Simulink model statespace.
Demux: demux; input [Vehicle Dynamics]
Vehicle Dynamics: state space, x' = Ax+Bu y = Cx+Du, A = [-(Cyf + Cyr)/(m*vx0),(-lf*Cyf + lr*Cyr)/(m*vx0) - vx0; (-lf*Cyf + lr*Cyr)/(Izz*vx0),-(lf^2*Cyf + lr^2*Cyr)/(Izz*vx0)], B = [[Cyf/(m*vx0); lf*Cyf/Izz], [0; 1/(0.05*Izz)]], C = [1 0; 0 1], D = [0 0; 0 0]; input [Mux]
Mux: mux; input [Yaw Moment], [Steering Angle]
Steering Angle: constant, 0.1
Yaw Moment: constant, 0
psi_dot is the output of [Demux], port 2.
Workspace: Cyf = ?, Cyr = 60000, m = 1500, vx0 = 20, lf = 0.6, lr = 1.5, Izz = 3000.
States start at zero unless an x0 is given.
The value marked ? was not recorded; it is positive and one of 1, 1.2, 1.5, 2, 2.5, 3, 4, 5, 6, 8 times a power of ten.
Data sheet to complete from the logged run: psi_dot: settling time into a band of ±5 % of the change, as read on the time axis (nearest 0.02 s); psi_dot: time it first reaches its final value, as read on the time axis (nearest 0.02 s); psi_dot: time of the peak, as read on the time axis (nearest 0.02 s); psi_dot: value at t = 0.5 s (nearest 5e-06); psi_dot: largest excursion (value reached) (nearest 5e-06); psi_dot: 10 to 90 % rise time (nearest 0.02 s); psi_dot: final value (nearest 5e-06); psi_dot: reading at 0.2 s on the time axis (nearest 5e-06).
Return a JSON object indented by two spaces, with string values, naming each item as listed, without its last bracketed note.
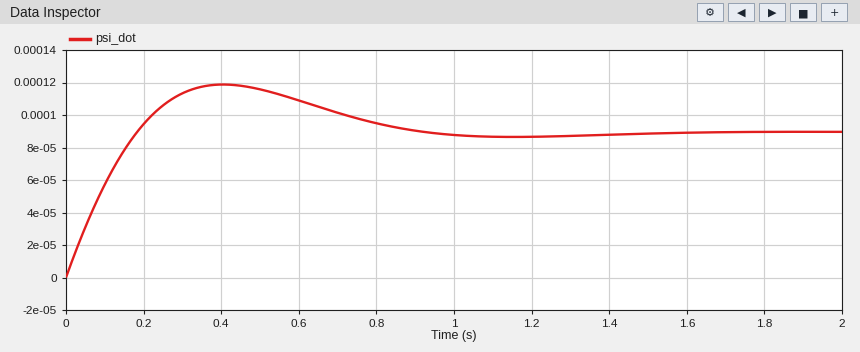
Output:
{
  "psi_dot: settling time into a band of ±5 % of the change, as read on the time axis": "0.82 s",
  "psi_dot: time it first reaches its final value, as read on the time axis": "0.18 s",
  "psi_dot: time of the peak, as read on the time axis": "0.40 s",
  "psi_dot: value at t = 0.5 s": "0.000115",
  "psi_dot: largest excursion (value reached)": "0.000120",
  "psi_dot: 10 to 90 % rise time": "0.14 s",
  "psi_dot: final value": "0.000090",
  "psi_dot: reading at 0.2 s on the time axis": "0.000095"
}
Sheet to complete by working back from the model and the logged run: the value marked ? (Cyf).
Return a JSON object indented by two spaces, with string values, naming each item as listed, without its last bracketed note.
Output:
{
  "the value marked ?": "50000"
}
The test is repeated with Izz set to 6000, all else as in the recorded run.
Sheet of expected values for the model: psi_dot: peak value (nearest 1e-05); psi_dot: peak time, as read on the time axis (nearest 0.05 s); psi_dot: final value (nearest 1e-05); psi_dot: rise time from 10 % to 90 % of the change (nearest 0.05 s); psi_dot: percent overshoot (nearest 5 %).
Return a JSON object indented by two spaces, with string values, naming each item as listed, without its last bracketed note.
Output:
{
  "psi_dot: peak value": "0.00010",
  "psi_dot: peak time, as read on the time axis": "0.70 s",
  "psi_dot: final value": "0.00009",
  "psi_dot: rise time from 10 % to 90 % of the change": "0.30 s",
  "psi_dot: percent overshoot": "15 %"
}
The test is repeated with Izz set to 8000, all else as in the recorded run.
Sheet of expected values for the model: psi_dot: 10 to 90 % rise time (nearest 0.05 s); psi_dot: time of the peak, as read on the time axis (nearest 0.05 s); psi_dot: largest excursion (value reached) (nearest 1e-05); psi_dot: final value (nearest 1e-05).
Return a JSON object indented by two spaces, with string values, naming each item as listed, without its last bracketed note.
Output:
{
  "psi_dot: 10 to 90 % rise time": "0.45 s",
  "psi_dot: time of the peak, as read on the time axis": "0.95 s",
  "psi_dot: largest excursion (value reached)": "0.00010",
  "psi_dot: final value": "0.00009"
}
